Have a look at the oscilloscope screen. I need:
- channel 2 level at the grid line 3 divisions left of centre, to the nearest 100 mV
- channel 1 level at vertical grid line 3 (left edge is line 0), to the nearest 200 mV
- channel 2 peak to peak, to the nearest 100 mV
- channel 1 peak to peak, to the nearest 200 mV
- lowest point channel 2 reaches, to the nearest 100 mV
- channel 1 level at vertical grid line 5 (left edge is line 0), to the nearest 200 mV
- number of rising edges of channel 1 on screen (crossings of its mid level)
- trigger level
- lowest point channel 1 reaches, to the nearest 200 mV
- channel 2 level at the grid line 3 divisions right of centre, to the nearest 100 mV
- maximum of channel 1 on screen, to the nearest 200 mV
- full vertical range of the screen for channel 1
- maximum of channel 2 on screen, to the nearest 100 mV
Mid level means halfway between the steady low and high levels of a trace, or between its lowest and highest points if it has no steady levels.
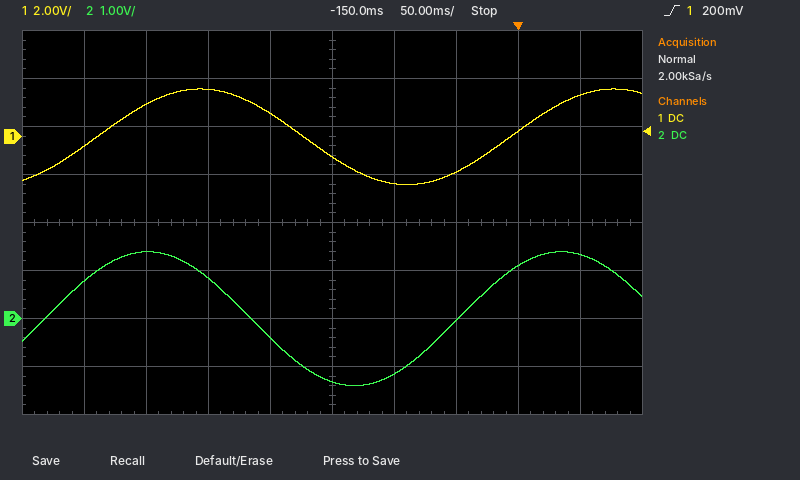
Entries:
1.4 V
2.0 V
2.8 V
4.0 V
-1.4 V
-800 mV
2
200 mV
-2.0 V
1.1 V
2.0 V
16 V
1.4 V
